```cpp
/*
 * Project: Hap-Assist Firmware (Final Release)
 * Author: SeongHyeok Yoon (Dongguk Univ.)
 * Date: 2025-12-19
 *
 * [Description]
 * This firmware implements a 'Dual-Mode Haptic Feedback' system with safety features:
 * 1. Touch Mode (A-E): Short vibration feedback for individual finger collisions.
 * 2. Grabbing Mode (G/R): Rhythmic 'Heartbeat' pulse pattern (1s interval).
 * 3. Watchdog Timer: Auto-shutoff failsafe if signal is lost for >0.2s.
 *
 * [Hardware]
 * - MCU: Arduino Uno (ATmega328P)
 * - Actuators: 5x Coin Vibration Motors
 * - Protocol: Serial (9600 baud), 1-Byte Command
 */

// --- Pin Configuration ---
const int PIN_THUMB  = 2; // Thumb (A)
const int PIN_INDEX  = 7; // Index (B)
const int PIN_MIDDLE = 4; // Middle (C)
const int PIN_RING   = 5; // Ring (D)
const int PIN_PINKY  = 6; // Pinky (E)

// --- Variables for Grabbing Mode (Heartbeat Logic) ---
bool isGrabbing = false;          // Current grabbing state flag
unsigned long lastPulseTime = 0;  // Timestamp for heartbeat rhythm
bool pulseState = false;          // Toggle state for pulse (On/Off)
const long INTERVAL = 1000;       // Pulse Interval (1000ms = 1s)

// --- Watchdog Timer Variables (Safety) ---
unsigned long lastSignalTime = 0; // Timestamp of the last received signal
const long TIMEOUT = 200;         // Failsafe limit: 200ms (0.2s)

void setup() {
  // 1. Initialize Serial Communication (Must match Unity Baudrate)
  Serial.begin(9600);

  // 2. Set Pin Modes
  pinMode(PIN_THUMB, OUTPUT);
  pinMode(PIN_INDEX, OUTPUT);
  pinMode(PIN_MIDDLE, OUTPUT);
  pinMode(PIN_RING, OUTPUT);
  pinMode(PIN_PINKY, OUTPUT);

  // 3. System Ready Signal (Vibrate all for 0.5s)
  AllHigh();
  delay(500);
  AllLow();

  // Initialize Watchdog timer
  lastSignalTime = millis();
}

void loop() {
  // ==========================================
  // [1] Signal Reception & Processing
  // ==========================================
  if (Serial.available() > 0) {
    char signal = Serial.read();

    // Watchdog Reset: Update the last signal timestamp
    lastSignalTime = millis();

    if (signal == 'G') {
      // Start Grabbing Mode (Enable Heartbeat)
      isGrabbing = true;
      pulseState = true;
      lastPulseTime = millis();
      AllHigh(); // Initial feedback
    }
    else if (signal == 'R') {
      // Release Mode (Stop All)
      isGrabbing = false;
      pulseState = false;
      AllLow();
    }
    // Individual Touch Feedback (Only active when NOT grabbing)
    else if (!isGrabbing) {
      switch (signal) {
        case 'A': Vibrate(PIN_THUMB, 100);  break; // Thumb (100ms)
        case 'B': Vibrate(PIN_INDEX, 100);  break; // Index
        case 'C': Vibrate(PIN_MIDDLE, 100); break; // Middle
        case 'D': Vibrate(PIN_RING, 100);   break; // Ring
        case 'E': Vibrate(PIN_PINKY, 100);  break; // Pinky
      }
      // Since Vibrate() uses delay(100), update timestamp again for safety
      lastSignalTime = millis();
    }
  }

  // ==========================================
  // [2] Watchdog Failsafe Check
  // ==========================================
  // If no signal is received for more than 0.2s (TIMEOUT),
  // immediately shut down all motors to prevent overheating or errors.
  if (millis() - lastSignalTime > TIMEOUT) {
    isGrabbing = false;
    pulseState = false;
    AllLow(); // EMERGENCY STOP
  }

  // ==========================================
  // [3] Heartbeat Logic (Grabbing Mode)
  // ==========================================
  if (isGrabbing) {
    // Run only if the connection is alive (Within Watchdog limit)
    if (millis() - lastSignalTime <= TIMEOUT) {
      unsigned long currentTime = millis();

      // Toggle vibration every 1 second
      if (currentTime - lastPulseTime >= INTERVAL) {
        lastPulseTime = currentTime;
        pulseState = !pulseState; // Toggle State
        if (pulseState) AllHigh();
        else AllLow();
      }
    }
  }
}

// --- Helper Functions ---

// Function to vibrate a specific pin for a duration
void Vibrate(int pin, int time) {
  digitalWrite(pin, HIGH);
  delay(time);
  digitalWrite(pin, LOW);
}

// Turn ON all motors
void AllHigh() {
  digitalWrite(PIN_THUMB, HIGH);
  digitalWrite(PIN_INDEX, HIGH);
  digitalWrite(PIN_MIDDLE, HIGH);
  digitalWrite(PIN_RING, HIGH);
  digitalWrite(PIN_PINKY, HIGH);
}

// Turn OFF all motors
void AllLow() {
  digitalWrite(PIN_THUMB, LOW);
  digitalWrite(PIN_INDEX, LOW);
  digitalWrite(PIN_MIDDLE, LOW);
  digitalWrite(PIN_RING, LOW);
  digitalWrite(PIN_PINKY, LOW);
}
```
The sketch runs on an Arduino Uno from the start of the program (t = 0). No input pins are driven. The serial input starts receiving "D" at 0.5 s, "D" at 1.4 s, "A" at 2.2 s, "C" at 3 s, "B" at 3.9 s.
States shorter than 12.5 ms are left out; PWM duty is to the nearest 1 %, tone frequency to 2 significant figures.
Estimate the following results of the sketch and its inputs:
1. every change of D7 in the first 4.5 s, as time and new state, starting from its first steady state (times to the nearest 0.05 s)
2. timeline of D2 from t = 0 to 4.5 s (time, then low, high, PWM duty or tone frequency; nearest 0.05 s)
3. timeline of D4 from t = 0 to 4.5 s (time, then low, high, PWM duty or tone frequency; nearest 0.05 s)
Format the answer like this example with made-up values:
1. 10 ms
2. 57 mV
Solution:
1. 0 s high; 0.5 s low; 3.9 s high; 4 s low
2. 0 s high; 0.5 s low; 2.2 s high; 2.3 s low
3. 0 s high; 0.5 s low; 3 s high; 3.1 s low
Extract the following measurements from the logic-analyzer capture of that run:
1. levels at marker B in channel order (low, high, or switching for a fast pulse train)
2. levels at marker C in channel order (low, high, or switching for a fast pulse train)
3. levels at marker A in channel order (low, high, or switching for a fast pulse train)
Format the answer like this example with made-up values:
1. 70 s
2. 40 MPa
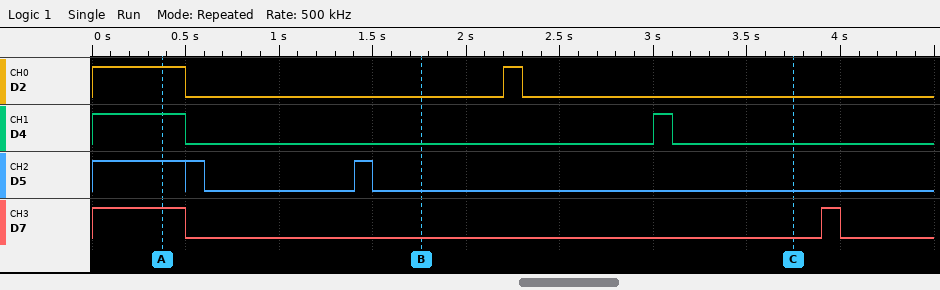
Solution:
1. D2 low, D4 low, D5 low, D7 low
2. D2 low, D4 low, D5 low, D7 low
3. D2 high, D4 high, D5 high, D7 high
